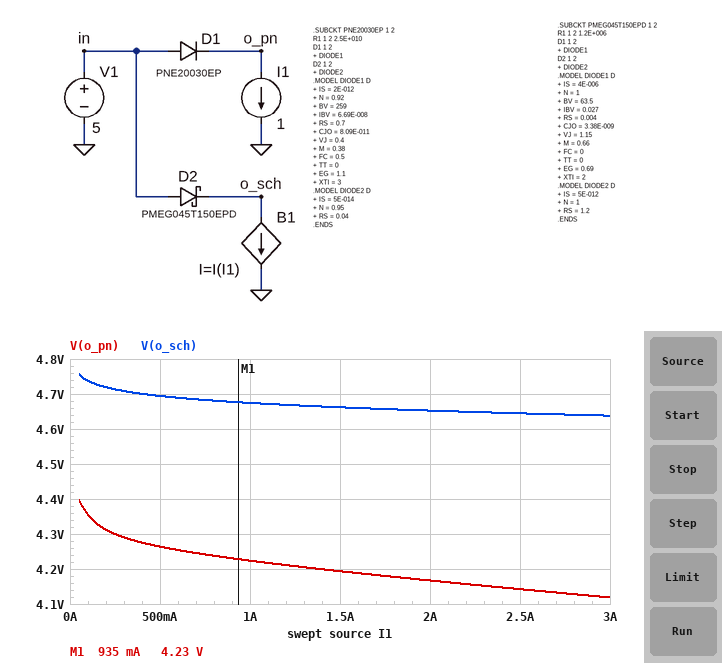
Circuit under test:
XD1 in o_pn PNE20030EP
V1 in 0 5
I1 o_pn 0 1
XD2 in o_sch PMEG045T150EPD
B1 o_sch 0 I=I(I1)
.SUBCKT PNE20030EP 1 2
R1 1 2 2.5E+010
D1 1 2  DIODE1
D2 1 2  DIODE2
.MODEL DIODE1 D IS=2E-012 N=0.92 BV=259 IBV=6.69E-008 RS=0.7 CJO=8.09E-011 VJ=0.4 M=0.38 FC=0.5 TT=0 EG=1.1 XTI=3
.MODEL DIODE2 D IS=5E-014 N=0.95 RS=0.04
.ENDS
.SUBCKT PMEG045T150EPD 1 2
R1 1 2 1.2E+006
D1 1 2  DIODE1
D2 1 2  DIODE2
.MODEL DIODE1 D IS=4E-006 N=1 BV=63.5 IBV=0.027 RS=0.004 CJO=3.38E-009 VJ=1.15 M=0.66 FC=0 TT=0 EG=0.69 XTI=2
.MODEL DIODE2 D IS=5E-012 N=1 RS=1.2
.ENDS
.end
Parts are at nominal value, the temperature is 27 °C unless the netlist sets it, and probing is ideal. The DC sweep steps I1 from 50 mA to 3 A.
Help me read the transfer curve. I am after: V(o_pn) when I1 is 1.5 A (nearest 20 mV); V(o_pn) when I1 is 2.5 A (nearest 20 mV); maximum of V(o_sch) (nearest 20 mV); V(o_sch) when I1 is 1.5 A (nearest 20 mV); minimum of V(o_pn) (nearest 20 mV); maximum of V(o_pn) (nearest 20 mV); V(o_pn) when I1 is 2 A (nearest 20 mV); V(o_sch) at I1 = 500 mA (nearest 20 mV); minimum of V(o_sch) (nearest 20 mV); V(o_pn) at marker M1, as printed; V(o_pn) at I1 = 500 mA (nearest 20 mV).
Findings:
4.20 V
4.14 V
4.76 V
4.66 V
4.12 V
4.40 V
4.16 V
4.70 V
4.64 V
4.23 V
4.26 V
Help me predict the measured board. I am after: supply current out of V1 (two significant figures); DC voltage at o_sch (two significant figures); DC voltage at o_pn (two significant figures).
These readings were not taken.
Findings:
2.0 A
4.7 V
4.2 V
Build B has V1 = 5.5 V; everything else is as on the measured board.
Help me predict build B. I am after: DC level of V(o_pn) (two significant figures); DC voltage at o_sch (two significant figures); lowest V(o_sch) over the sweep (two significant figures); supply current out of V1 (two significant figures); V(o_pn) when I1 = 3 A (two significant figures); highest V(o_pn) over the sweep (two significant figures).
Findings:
4.7 V
5.2 V
5.1 V
2.0 A
4.6 V
4.9 V
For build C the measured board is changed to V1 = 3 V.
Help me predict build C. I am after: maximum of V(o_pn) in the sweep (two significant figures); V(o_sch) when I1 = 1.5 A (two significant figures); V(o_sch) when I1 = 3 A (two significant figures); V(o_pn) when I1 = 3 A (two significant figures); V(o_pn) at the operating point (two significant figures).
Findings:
2.4 V
2.7 V
2.6 V
2.1 V
2.2 V
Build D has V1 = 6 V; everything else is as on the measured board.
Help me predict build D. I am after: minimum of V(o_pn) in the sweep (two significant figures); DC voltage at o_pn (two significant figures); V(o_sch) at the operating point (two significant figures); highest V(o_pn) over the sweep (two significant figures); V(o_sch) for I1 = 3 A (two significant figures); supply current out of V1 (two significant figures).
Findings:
5.1 V
5.2 V
5.7 V
5.4 V
5.6 V
2.0 A
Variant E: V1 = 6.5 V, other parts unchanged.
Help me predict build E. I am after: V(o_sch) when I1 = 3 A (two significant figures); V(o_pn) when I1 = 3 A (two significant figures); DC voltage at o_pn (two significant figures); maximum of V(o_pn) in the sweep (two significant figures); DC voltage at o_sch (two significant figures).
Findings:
6.1 V
5.6 V
5.7 V
5.9 V
6.2 V
